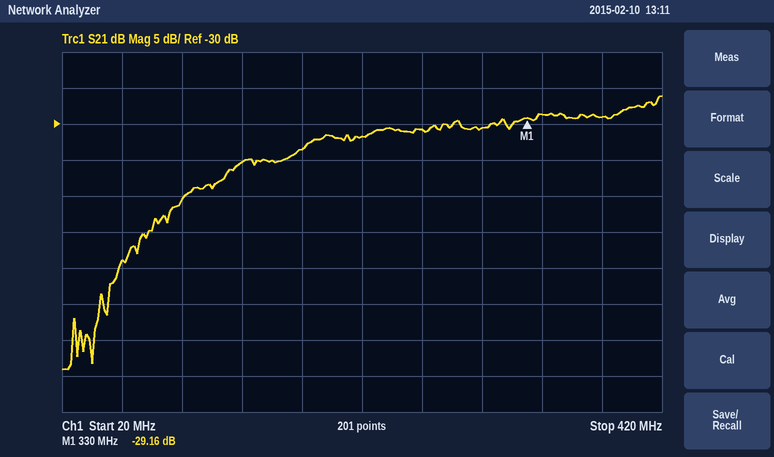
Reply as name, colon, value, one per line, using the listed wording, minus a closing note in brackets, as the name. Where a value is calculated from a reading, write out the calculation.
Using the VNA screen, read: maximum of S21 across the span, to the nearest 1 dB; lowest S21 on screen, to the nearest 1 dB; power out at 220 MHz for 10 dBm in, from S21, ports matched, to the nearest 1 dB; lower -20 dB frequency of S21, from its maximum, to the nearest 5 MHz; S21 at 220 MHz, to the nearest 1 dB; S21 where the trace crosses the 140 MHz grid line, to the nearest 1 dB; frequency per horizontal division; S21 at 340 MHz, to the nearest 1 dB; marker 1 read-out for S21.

maximum of S21 across the span, to the nearest 1 dB: -26 dB
lowest S21 on screen, to the nearest 1 dB: -64 dB
power out at 220 MHz for 10 dBm in, from S21, ports matched, to the nearest 1 dB: 10 dBm + (-32 dB) = -22 dBm
lower -20 dB frequency of S21, from its maximum, to the nearest 5 MHz: 70 MHz
S21 at 220 MHz, to the nearest 1 dB: -32 dB
S21 where the trace crosses the 140 MHz grid line, to the nearest 1 dB: -35 dB
frequency per horizontal division: 40 MHz
S21 at 340 MHz, to the nearest 1 dB: -29 dB
marker 1 read-out for S21: -29.16 dB
